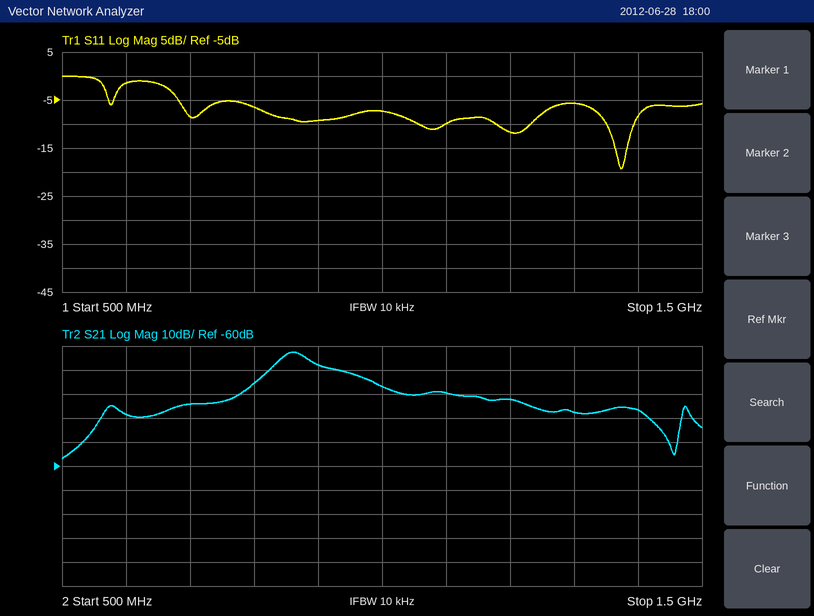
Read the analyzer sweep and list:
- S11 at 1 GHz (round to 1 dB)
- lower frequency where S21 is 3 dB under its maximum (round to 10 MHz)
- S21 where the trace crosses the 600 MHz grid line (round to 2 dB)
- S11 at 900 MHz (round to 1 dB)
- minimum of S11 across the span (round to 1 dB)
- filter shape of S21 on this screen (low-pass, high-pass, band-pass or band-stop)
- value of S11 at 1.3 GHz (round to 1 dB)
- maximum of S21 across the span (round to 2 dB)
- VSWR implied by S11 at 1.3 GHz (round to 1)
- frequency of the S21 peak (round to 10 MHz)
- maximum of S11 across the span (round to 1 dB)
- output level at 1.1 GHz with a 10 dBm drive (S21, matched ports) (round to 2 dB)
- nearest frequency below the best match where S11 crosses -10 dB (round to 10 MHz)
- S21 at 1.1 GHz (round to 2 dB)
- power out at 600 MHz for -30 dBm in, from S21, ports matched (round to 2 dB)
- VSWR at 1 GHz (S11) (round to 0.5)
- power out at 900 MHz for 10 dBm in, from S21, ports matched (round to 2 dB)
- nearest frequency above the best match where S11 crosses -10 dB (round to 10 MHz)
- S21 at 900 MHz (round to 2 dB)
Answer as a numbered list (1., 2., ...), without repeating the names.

1. -7 dB
2. 840 MHz
3. -38 dB
4. -9 dB
5. -19 dB
6. band-pass
7. -6 dB
8. -12 dB
9. 3
10. 860 MHz
11. 0 dB
12. -20 dBm
13. 1.35 GHz
14. -30 dB
15. -68 dBm
16. 2.5
17. -8 dBm
18. 1.39 GHz
19. -18 dB
